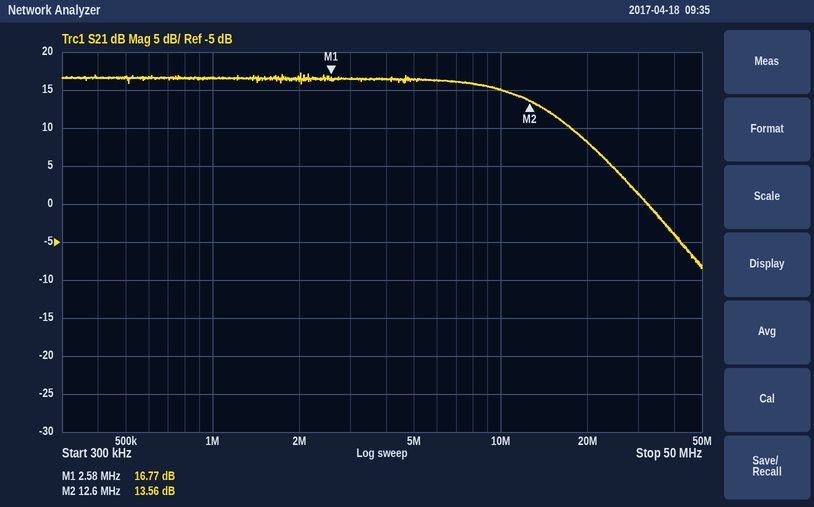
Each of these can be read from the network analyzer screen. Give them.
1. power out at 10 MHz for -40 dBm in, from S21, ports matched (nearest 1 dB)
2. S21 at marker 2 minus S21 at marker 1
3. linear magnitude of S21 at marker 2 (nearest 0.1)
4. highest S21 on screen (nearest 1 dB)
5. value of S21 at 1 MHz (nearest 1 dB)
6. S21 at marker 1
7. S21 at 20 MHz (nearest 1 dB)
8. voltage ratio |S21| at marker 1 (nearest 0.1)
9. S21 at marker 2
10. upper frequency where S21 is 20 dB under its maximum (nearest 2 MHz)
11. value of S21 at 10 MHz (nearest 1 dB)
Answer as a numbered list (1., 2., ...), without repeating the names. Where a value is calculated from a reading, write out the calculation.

1. -40 dBm + (15 dB) = -25 dBm
2. 13.56 − (16.77) = -3.21 dB
3. 10^(13.56/20) ≈ 4.8
4. 17 dB
5. 17 dB
6. 16.77 dB
7. 8 dB
8. 10^(16.77/20) ≈ 6.9
9. 13.56 dB
10. 38 MHz
11. 15 dB
